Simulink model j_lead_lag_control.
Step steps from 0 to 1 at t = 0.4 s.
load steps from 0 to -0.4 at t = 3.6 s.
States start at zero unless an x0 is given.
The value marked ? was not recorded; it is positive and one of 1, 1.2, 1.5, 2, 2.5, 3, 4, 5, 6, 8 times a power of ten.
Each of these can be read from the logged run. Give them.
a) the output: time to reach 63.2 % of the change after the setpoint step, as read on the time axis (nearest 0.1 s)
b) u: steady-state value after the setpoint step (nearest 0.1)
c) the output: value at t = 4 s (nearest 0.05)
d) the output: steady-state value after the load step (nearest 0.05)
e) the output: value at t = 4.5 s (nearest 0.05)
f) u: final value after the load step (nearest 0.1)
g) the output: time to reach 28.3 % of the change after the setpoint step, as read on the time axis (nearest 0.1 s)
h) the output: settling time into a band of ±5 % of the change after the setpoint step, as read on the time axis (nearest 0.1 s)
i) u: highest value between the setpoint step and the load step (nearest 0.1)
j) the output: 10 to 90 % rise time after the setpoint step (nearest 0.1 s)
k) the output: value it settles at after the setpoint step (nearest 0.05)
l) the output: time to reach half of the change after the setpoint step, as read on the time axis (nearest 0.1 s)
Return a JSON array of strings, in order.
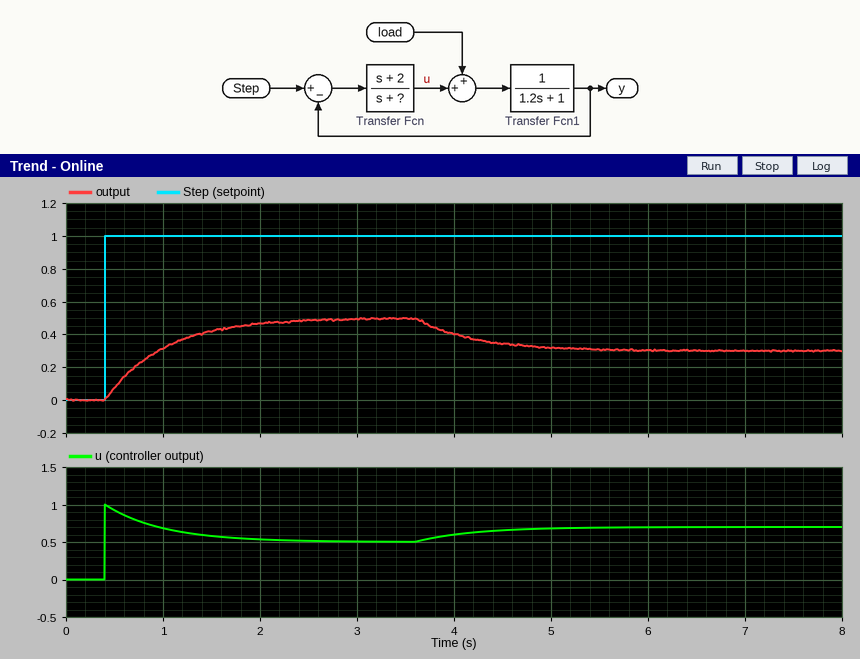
["1.0 s", "0.5", "0.40", "0.30", "0.35", "0.7", "0.6 s", "2.2 s", "1.0", "1.3 s", "0.50", "0.8 s"]
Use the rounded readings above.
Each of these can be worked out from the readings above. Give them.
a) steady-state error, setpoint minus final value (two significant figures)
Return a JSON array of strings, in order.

["0.50"]
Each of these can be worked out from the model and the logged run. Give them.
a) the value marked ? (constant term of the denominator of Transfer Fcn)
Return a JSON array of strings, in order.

["2"]
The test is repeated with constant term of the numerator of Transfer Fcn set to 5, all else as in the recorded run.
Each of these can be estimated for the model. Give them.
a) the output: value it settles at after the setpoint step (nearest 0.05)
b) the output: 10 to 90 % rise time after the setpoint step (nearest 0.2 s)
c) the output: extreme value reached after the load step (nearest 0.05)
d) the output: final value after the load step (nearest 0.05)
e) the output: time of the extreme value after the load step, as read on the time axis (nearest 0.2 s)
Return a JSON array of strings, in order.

["0.70", "0.8 s", "0.60", "0.60", "4.6 s"]
